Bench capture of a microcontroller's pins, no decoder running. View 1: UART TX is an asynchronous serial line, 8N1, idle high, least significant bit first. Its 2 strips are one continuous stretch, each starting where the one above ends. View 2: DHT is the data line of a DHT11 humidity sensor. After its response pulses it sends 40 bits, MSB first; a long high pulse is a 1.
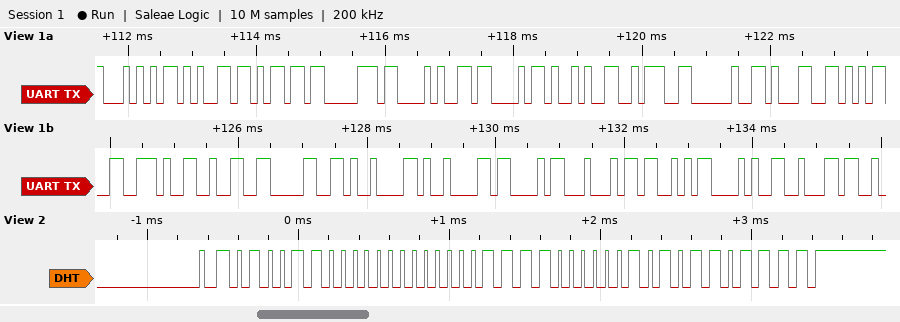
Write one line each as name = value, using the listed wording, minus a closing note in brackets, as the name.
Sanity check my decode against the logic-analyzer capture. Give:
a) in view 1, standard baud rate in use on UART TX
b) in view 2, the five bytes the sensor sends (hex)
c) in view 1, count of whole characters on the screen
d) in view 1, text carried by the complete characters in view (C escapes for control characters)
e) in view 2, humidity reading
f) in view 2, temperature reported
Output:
in view 1, standard baud rate in use on UART TX = 9600 baud
in view 2, the five bytes the sensor sends = 4C 00 1E 05 6F
in view 1, count of whole characters on the screen = 21
in view 1, text carried by the complete characters in view = "Temp(C): 15.20\t\tCDS(b"
in view 2, humidity reading = 76 %
in view 2, temperature reported = 30.5 °C
